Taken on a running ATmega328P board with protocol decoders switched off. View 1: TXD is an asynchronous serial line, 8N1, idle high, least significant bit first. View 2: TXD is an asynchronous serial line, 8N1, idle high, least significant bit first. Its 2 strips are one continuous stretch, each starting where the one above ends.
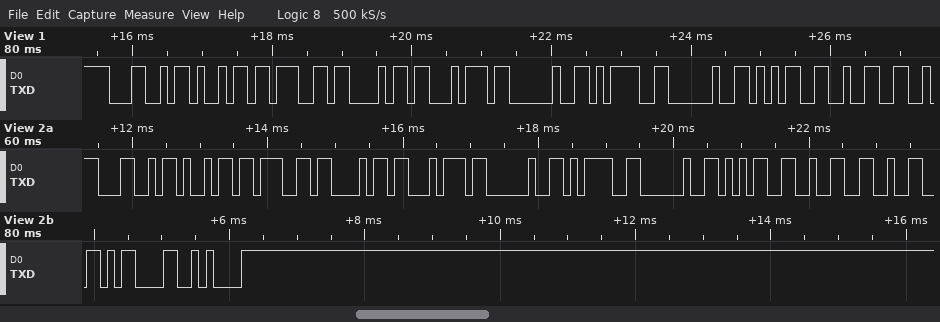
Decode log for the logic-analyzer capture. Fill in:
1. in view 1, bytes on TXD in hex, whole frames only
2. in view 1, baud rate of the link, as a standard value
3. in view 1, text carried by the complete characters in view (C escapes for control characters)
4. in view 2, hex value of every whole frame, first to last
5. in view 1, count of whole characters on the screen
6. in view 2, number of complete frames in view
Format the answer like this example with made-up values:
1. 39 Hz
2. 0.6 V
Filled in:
1. 4C 69 67 68 74 20 3D 20 35 32
2. 9600 baud
3. "Light = 52"
4. 4C 69 67 68 74 20 3D 20 35 32 32 0D 0A
5. 10
6. 13
